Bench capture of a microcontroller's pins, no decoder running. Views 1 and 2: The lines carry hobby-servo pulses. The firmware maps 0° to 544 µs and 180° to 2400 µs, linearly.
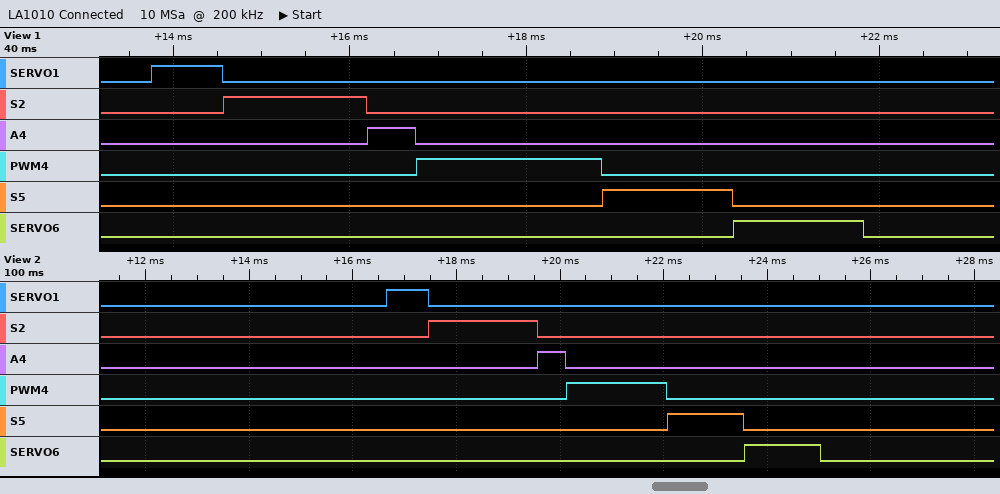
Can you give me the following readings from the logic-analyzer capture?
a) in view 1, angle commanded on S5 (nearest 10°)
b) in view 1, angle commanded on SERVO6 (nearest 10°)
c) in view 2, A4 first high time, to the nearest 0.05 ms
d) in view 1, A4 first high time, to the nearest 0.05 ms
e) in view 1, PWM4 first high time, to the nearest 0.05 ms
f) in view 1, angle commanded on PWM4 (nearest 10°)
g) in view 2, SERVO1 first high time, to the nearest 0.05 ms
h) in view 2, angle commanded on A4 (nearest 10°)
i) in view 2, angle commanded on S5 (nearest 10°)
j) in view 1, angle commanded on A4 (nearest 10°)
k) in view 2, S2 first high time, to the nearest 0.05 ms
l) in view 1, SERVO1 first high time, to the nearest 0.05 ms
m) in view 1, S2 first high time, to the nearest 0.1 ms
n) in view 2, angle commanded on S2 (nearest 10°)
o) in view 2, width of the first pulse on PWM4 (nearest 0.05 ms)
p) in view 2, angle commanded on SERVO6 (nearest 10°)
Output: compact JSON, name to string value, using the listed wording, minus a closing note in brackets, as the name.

{"in view 1, angle commanded on S5": "90°", "in view 1, angle commanded on SERVO6": "90°", "in view 2, A4 first high time, to the nearest 0.05 ms": "0.55 ms", "in view 1, A4 first high time, to the nearest 0.05 ms": "0.55 ms", "in view 1, PWM4 first high time, to the nearest 0.05 ms": "2.10 ms", "in view 1, angle commanded on PWM4": "150°", "in view 2, SERVO1 first high time, to the nearest 0.05 ms": "0.80 ms", "in view 2, angle commanded on A4": "0°", "in view 2, angle commanded on S5": "90°", "in view 1, angle commanded on A4": "0°", "in view 2, S2 first high time, to the nearest 0.05 ms": "2.10 ms", "in view 1, SERVO1 first high time, to the nearest 0.05 ms": "0.80 ms", "in view 1, S2 first high time, to the nearest 0.1 ms": "1.6 ms", "in view 2, angle commanded on S2": "150°", "in view 2, width of the first pulse on PWM4": "1.95 ms", "in view 2, angle commanded on SERVO6": "90°"}
